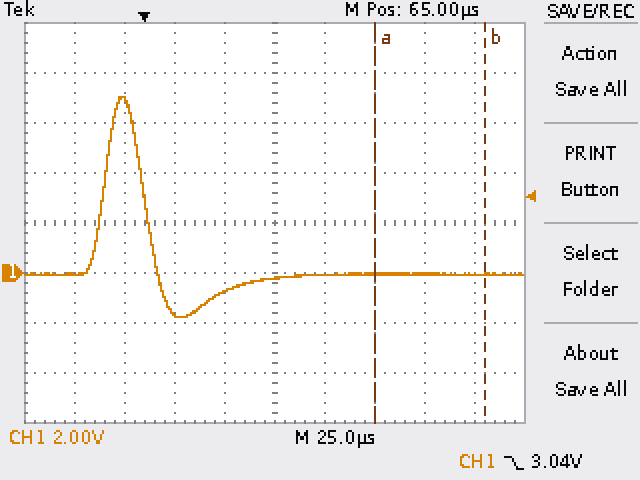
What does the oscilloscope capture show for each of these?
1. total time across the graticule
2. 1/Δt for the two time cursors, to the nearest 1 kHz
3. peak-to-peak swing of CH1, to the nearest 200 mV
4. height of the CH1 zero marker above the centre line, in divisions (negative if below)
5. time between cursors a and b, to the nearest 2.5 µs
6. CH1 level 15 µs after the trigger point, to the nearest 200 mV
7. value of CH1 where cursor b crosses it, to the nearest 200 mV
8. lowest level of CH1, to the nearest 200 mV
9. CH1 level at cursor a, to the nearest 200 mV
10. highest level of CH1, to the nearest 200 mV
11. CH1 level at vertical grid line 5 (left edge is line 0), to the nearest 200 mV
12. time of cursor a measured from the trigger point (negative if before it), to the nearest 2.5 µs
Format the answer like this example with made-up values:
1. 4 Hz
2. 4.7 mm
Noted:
1. 250 µs
2. 18 kHz
3. 8.8 V
4. -1.0 div
5. 55.0 µs
6. -1.6 V
7. 0.0 V
8. -1.8 V
9. 0.0 V
10. 7.0 V
11. -200 mV
12. +115.0 µs
